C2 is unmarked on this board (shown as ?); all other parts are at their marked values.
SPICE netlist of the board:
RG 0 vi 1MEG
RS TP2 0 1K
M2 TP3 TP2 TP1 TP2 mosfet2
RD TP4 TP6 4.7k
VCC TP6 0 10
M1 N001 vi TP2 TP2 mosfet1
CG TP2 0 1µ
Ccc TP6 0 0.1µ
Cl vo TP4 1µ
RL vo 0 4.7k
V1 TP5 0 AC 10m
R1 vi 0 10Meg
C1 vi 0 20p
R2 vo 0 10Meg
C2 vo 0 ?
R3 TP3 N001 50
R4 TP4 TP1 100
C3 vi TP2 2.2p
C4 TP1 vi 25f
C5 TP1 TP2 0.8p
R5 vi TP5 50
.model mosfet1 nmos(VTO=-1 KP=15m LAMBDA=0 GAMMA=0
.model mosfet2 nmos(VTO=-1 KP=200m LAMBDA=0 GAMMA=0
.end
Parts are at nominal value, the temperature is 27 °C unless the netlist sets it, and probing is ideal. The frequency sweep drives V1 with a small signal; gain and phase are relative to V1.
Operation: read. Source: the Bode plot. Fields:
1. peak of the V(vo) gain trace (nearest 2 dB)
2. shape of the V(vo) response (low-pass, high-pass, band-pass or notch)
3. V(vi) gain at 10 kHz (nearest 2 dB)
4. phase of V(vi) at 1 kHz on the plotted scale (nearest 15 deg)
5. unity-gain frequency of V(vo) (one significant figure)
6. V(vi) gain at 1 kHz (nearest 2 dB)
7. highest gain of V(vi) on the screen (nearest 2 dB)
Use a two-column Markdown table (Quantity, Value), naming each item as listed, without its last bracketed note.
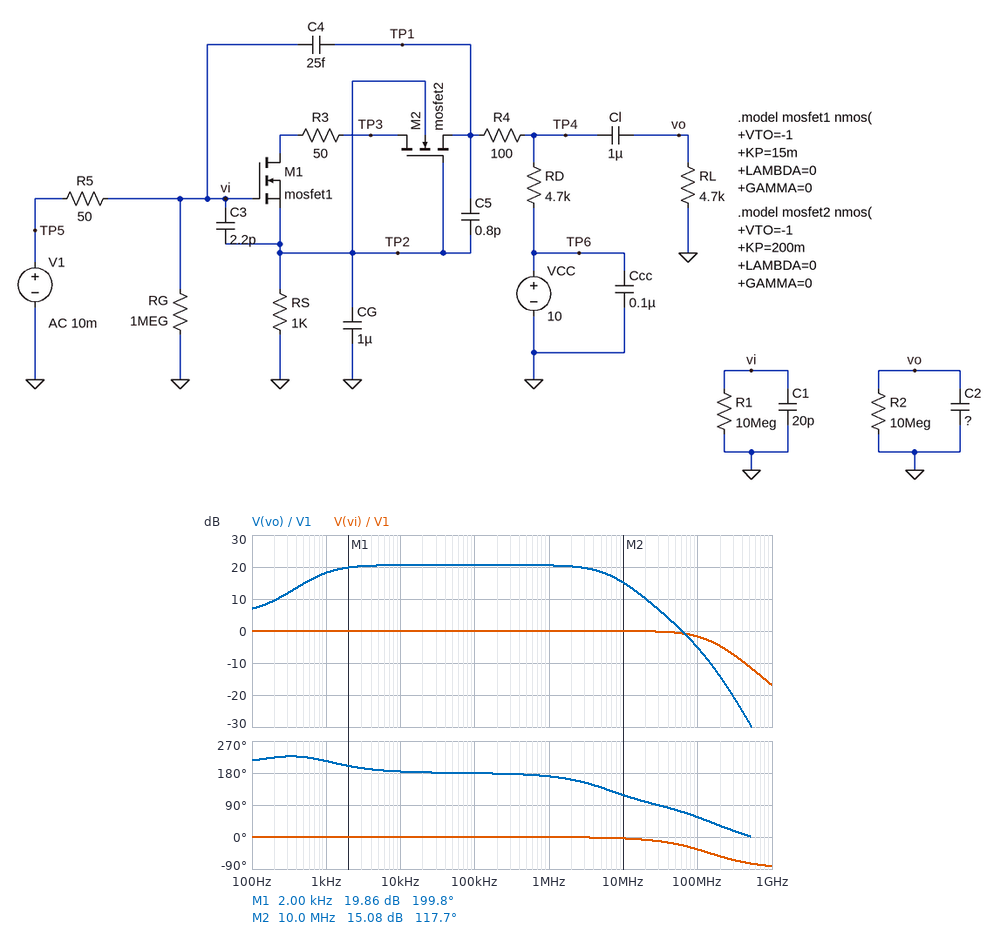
| Quantity | Value |
|---|---|
| peak of the V(vo) gain trace | 20 dB |
| shape of the V(vo) response | band-pass |
| V(vi) gain at 10 kHz | 0 dB |
| phase of V(vi) at 1 kHz on the plotted scale | 0 deg |
| unity-gain frequency of V(vo) | 60 MHz |
| V(vi) gain at 1 kHz | 0 dB |
| highest gain of V(vi) on the screen | 0 dB |
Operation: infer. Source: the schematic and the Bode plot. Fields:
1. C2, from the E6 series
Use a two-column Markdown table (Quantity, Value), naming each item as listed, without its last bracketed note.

| Quantity | Value |
|---|---|
| C2, from the E6 series | 10 pF |
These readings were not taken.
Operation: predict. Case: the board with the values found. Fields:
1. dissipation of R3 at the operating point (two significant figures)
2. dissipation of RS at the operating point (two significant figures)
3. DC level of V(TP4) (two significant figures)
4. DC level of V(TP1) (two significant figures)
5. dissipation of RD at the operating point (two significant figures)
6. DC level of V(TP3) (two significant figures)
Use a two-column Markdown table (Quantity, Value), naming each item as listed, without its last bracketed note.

| Quantity | Value |
|---|---|
| dissipation of R3 at the operating point | 24 µW |
| dissipation of RS at the operating point | 480 µW |
| DC level of V(TP4) | 6.7 V |
| DC level of V(TP1) | 6.7 V |
| dissipation of RD at the operating point | 2.3 mW |
| DC level of V(TP3) | 1.6 V |
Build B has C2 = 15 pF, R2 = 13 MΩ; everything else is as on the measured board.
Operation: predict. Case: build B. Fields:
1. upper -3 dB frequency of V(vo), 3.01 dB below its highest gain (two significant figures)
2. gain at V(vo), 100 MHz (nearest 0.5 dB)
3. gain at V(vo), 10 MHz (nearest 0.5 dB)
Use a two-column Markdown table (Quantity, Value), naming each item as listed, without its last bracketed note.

| Quantity | Value |
|---|---|
| upper -3 dB frequency of V(vo), 3.01 dB below its highest gain | 4.3 MHz |
| gain at V(vo), 100 MHz | -8.5 dB |
| gain at V(vo), 10 MHz | 12.5 dB |
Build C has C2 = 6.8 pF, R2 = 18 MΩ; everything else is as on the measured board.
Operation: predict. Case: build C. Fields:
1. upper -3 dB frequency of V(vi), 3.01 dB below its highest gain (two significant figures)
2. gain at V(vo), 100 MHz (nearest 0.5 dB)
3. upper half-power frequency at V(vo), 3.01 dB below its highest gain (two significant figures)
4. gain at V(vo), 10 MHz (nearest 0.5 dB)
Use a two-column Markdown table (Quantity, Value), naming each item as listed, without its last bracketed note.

| Quantity | Value |
|---|---|
| upper -3 dB frequency of V(vi), 3.01 dB below its highest gain | 140 MHz |
| gain at V(vo), 100 MHz | -2.0 dB |
| upper half-power frequency at V(vo), 3.01 dB below its highest gain | 8.8 MHz |
| gain at V(vo), 10 MHz | 17.0 dB |
